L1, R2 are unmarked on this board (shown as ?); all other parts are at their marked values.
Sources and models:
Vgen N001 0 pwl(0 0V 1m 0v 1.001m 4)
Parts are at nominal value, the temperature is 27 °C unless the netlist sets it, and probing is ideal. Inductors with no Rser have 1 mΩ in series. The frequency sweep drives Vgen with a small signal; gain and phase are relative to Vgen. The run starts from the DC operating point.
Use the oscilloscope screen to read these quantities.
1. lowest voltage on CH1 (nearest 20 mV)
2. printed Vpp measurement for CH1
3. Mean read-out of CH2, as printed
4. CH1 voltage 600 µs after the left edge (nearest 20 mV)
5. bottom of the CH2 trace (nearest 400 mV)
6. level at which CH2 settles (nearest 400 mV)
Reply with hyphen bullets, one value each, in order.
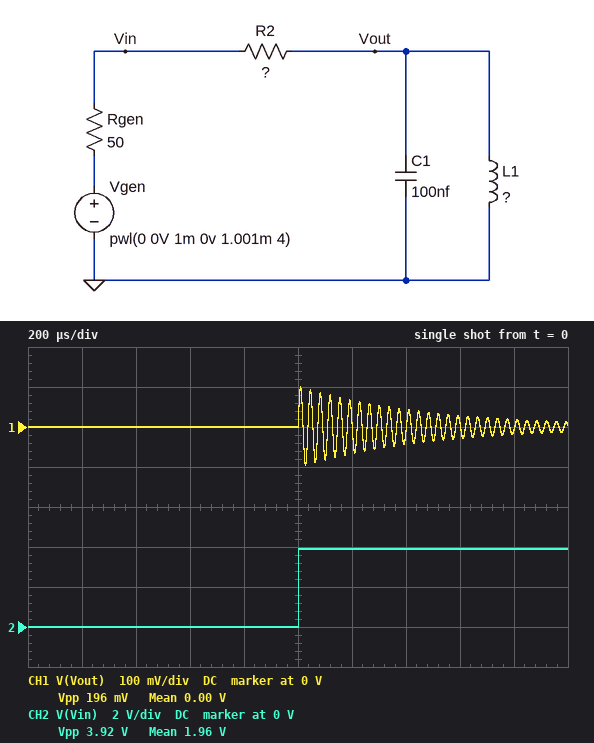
- -100 mV
- 196 mV
- 1.96 V
- 0 V
- 0 V
- 4.0 V
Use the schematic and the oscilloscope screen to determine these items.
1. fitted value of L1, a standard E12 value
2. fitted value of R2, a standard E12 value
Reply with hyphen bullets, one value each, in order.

- 330 µH
- 2.2 kΩ
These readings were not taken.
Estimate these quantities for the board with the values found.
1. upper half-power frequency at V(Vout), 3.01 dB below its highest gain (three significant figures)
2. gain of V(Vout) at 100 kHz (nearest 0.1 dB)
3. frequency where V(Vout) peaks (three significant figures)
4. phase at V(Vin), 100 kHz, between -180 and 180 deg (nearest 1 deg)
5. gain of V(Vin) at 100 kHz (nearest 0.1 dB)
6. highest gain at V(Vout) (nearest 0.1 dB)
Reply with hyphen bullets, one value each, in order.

- 28.1 kHz
- -42.3 dB
- 27.7 kHz
- 0 deg
- -0.2 dB
- 0 dB
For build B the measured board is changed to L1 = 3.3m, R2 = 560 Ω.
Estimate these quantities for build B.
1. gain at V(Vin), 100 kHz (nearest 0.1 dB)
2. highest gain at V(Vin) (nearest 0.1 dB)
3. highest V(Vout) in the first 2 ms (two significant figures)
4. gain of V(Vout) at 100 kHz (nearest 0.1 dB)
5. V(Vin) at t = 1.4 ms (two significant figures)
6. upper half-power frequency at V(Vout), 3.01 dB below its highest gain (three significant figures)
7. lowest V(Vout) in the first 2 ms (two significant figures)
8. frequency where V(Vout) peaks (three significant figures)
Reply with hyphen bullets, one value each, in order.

- -0.7 dB
- 0 dB
- 960 mV
- -31.6 dB
- 3.7 V
- 10.2 kHz
- -600 mV
- 8.76 kHz
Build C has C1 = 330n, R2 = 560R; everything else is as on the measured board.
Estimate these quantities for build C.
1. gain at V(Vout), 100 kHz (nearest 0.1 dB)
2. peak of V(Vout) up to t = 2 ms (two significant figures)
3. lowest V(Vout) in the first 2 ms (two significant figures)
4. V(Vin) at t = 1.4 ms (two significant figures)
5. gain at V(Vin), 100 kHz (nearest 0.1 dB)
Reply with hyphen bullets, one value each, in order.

- -41.8 dB
- 200 mV
- -180 mV
- 3.7 V
- -0.7 dB
